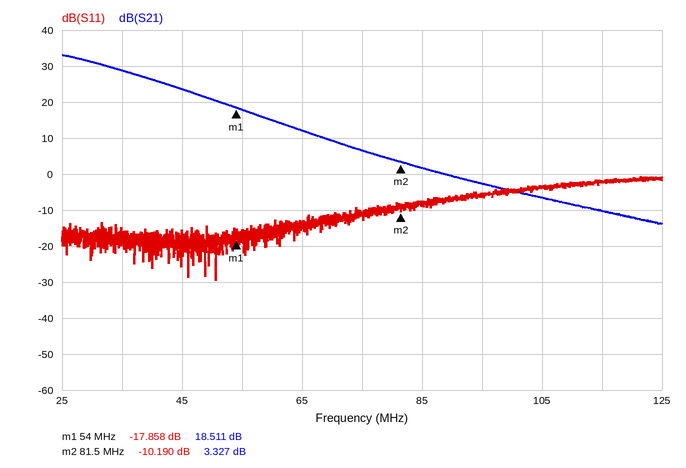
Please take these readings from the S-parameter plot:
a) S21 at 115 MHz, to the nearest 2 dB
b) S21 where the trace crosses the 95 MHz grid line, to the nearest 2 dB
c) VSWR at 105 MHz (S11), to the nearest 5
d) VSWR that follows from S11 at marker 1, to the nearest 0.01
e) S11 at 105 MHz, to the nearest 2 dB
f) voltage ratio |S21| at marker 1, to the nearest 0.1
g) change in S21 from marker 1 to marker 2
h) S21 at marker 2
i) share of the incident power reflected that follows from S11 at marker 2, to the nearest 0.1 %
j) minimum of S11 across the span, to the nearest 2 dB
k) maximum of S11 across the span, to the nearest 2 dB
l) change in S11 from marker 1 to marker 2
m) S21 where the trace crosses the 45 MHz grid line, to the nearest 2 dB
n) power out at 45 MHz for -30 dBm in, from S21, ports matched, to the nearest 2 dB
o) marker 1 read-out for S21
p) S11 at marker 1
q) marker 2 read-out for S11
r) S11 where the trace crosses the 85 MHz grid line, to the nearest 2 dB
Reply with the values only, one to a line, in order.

-10 dB
-2 dB
5
1.29
-4 dB
8.4
-15.184 dB
3.327 dB
9.6 %
-30 dB
0 dB
7.668 dB
24 dB
-6 dBm
18.511 dB
-17.858 dB
-10.190 dB
-8 dB
